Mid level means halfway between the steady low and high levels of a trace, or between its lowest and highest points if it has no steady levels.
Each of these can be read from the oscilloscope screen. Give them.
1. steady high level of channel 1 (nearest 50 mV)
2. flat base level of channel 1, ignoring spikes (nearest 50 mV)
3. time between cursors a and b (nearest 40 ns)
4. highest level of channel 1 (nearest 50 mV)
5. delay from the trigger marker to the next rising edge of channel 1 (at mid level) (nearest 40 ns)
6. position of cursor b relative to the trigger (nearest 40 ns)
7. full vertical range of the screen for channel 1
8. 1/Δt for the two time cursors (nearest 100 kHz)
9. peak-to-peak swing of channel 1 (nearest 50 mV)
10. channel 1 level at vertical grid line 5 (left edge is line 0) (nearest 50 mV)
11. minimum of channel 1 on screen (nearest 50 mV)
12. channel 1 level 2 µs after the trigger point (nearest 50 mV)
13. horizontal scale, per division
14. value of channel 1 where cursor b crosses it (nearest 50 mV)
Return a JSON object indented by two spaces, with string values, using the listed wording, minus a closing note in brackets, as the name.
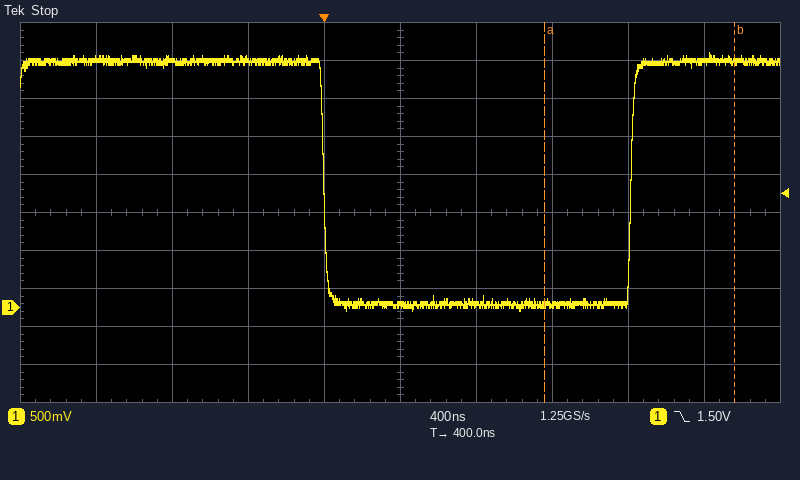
{
  "steady high level of channel 1": "3.25 V",
  "flat base level of channel 1, ignoring spikes": "50 mV",
  "time between cursors a and b": "1.00 µs",
  "highest level of channel 1": "3.35 V",
  "delay from the trigger marker to the next rising edge of channel 1 (at mid level)": "1.60 µs",
  "position of cursor b relative to the trigger": "+2.16 µs",
  "full vertical range of the screen for channel 1": "5 V",
  "1/Δt for the two time cursors": "1.0 MHz",
  "peak-to-peak swing of channel 1": "3.40 V",
  "channel 1 level at vertical grid line 5 (left edge is line 0)": "50 mV",
  "minimum of channel 1 on screen": "-50 mV",
  "channel 1 level 2 µs after the trigger point": "3.25 V",
  "horizontal scale, per division": "400 ns",
  "value of channel 1 where cursor b crosses it": "3.25 V"
}
